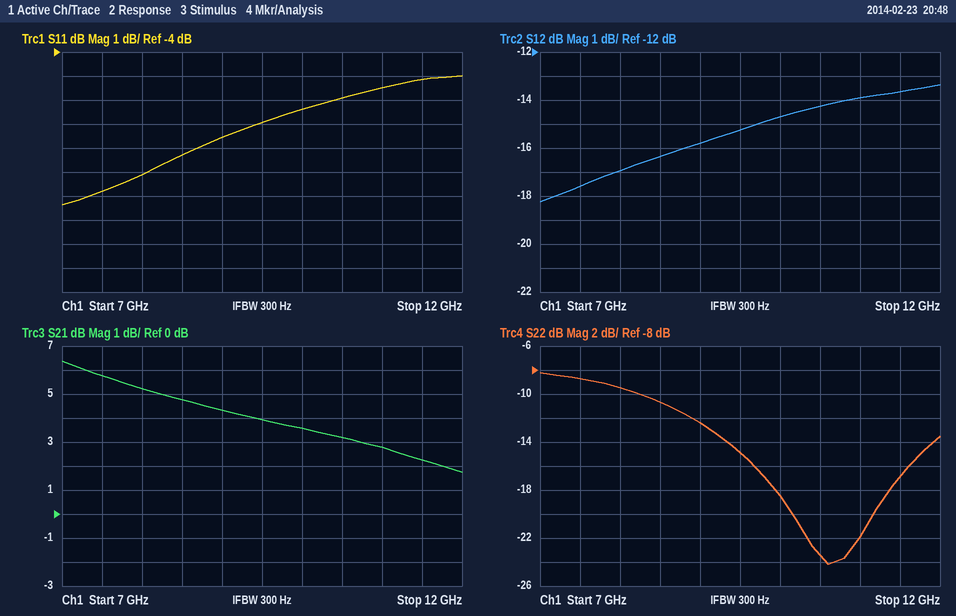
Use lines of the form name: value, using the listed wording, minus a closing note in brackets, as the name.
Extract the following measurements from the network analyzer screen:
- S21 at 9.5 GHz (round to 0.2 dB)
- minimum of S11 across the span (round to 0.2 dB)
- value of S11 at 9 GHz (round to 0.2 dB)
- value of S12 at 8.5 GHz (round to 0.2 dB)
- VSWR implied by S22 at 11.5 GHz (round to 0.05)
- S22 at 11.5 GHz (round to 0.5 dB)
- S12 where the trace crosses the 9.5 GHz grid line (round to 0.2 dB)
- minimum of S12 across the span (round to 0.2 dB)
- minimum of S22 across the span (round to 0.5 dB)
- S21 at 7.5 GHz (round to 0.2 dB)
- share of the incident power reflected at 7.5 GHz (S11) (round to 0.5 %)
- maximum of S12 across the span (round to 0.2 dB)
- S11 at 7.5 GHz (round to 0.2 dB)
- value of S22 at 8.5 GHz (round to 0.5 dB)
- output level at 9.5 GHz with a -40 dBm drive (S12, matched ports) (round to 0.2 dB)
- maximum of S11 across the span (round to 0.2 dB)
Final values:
S21 at 9.5 GHz: 4.0 dB
minimum of S11 across the span: -10.4 dB
value of S11 at 9 GHz: -7.6 dB
value of S12 at 8.5 GHz: -16.4 dB
VSWR implied by S22 at 11.5 GHz: 1.35
S22 at 11.5 GHz: -17.0 dB
S12 where the trace crosses the 9.5 GHz grid line: -15.2 dB
minimum of S12 across the span: -18.2 dB
minimum of S22 across the span: -24.0 dB
S21 at 7.5 GHz: 5.8 dB
share of the incident power reflected at 7.5 GHz (S11): 10.5 %
maximum of S12 across the span: -13.4 dB
S11 at 7.5 GHz: -9.8 dB
value of S22 at 8.5 GHz: -10.5 dB
output level at 9.5 GHz with a -40 dBm drive (S12, matched ports): -55.2 dBm
maximum of S11 across the span: -5.0 dB
